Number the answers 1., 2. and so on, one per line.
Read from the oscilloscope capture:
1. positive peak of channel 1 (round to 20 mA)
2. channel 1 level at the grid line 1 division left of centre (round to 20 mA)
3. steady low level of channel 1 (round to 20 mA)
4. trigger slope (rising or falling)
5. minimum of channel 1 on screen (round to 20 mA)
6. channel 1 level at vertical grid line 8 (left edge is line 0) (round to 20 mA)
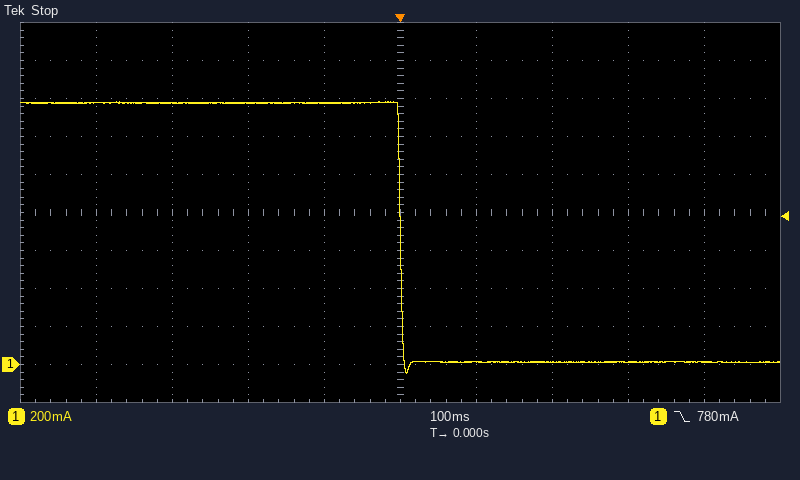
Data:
1. 1.38 A
2. 1.38 A
3. 20 mA
4. falling
5. -40 mA
6. 20 mA
